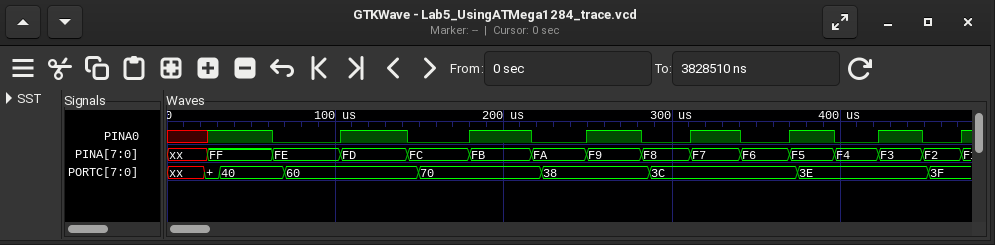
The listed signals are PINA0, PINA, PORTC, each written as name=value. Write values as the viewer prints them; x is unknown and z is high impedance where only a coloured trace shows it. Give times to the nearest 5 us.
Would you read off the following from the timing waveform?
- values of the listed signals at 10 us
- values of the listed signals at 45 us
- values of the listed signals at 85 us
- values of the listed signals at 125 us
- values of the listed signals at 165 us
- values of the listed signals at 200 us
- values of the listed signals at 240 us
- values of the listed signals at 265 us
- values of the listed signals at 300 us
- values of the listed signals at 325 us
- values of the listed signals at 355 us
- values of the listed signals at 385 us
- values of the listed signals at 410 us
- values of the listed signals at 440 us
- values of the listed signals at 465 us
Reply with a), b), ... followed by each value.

a) PINA0=x, PINA=xx, PORTC=xx
b) PINA0=1, PINA=FF, PORTC=40
c) PINA0=0, PINA=FE, PORTC=60
d) PINA0=1, PINA=FD, PORTC=60
e) PINA0=0, PINA=FC, PORTC=70
f) PINA0=1, PINA=FB, PORTC=70
g) PINA0=0, PINA=FA, PORTC=38
h) PINA0=1, PINA=F9, PORTC=38
i) PINA0=0, PINA=F8, PORTC=3C
j) PINA0=1, PINA=F7, PORTC=3C
k) PINA0=0, PINA=F6, PORTC=3C
l) PINA0=1, PINA=F5, PORTC=3E
m) PINA0=0, PINA=F4, PORTC=3E
n) PINA0=1, PINA=F3, PORTC=3E
o) PINA0=0, PINA=F2, PORTC=3F
